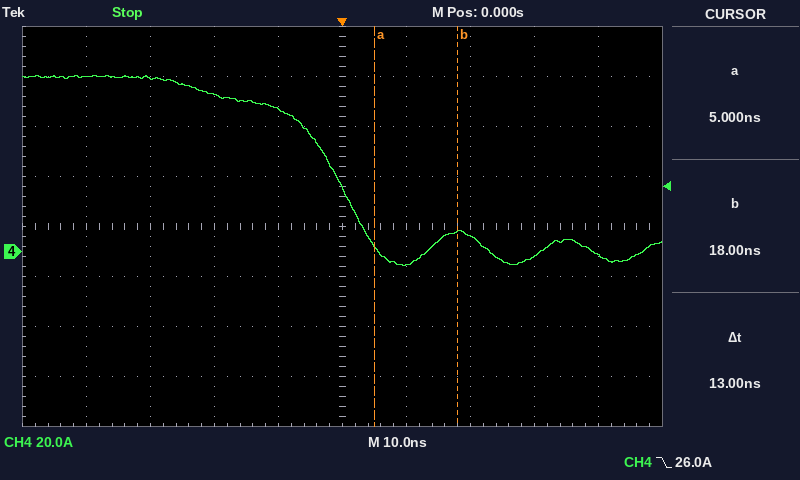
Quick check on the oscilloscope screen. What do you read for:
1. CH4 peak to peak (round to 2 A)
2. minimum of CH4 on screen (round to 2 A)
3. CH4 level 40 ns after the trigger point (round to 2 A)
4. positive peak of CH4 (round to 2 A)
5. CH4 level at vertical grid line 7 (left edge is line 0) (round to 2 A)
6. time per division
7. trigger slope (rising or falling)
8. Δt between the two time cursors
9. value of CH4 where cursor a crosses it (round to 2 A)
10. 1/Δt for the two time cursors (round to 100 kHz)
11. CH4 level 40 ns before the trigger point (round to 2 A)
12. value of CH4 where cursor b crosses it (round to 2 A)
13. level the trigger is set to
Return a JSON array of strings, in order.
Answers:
["76 A", "-6 A", "-2 A", "70 A", "6 A", "10 ns", "falling", "13 ns", "2 A", "76.9 MHz", "70 A", "8 A", "26.0 A"]
